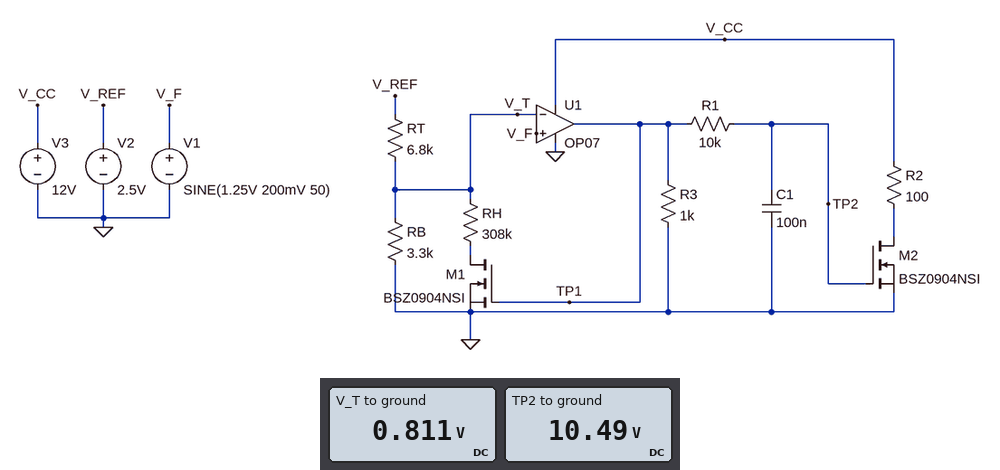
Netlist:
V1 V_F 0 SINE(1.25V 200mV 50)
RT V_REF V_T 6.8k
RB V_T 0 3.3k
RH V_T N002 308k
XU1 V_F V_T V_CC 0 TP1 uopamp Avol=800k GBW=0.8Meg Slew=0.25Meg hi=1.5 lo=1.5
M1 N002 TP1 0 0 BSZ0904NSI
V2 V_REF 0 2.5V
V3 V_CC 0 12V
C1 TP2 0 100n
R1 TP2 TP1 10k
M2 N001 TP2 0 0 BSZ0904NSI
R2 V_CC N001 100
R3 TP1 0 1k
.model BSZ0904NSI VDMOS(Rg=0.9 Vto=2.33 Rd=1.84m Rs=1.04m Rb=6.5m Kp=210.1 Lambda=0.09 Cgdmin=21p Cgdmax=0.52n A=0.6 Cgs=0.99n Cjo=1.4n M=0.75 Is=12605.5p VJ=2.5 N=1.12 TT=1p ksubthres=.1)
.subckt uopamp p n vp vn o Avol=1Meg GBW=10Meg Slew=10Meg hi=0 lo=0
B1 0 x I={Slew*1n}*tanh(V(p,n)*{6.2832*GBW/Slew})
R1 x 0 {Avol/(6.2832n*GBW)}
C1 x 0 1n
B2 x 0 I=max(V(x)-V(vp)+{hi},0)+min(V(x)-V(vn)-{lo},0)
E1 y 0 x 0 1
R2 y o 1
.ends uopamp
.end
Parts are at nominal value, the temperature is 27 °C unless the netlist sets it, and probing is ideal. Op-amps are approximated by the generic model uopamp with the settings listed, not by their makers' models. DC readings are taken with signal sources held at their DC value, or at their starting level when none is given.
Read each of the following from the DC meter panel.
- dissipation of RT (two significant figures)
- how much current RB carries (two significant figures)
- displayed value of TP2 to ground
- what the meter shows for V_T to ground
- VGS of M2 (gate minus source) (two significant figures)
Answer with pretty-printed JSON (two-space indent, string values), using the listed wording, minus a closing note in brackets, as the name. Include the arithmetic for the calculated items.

{
  "dissipation of RT": "(2.5 V - 811 mV)^2 / 6.8 kΩ = 420 µW",
  "how much current RB carries": "(811 mV) / 3.3 kΩ = 250 µA",
  "displayed value of TP2 to ground": "10.49 V",
  "what the meter shows for V_T to ground": "0.811 V",
  "VGS of M2 (gate minus source)": "10.49 V = 10 V"
}
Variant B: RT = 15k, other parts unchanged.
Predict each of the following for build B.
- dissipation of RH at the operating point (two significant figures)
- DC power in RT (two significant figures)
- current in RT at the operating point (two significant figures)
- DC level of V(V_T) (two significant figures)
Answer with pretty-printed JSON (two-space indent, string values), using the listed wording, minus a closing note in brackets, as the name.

{
  "dissipation of RH at the operating point": "650 nW",
  "DC power in RT": "280 µW",
  "current in RT at the operating point": "140 µA",
  "DC level of V(V_T)": "450 mV"
}
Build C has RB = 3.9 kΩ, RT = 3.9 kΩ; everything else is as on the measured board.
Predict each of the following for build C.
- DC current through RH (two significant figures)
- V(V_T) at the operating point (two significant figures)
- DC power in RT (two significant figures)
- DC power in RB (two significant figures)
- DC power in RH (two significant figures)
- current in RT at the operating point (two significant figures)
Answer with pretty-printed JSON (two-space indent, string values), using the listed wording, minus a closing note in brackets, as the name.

{
  "DC current through RH": "4.0 µA",
  "V(V_T) at the operating point": "1.2 V",
  "DC power in RT": "410 µW",
  "DC power in RB": "400 µW",
  "DC power in RH": "5.0 µW",
  "current in RT at the operating point": "320 µA"
}
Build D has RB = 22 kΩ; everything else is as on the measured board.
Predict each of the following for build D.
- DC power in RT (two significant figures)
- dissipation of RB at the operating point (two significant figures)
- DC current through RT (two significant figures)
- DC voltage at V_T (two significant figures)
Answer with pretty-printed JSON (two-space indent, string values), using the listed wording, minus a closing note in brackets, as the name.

{
  "DC power in RT": "51 µW",
  "dissipation of RB at the operating point": "170 µW",
  "DC current through RT": "87 µA",
  "DC voltage at V_T": "1.9 V"
}
